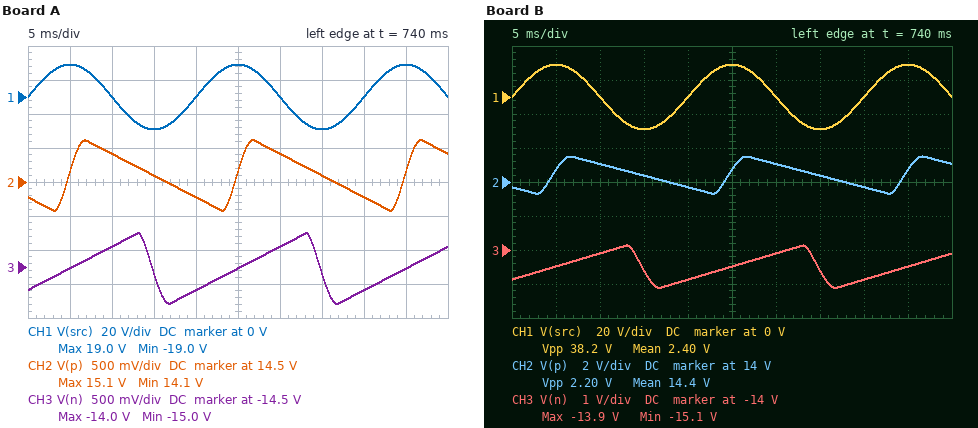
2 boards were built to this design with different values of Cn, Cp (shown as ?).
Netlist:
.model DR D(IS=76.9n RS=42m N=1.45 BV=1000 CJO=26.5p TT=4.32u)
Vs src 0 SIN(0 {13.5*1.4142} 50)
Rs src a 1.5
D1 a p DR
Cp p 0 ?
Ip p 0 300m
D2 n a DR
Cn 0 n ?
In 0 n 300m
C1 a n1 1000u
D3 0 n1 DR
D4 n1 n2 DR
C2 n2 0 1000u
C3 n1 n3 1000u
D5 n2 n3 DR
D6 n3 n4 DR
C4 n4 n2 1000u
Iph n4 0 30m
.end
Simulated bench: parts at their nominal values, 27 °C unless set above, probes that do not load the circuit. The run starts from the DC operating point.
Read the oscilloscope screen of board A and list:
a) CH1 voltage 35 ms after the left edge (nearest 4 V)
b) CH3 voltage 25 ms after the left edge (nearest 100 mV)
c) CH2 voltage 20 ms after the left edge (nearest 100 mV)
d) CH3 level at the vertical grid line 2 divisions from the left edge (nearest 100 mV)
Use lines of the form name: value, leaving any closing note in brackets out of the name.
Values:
CH1 voltage 35 ms after the left edge: -20 V
CH3 voltage 25 ms after the left edge: -14.5 V
CH2 voltage 20 ms after the left edge: 14.3 V
CH3 level at the vertical grid line 2 divisions from the left edge: -14.2 V
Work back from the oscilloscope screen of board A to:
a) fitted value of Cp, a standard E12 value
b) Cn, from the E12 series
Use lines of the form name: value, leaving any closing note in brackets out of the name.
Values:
fitted value of Cp, a standard E12 value: 4.7 mF
Cn, from the E12 series: 4.7 mF
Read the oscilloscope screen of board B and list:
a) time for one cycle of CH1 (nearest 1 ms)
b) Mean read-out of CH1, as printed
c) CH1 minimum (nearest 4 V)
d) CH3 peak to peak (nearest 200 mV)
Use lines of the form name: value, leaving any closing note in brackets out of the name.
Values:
time for one cycle of CH1: 20 ms
Mean read-out of CH1, as printed: 2.40 V
CH1 minimum: -20 V
CH3 peak to peak: 1.2 V
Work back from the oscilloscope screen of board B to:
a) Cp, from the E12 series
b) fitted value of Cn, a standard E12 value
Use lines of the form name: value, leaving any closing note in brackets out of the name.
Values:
Cp, from the E12 series: 2.2 mF
fitted value of Cn, a standard E12 value: 3.9 mF
